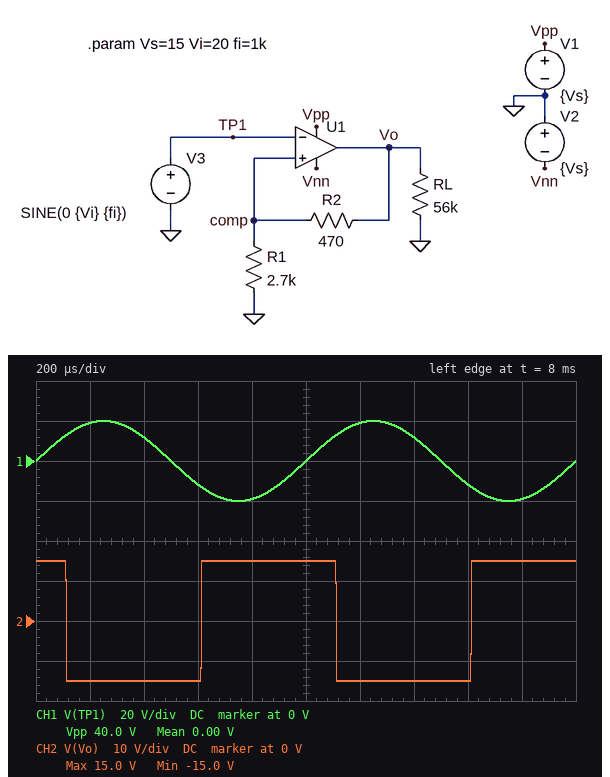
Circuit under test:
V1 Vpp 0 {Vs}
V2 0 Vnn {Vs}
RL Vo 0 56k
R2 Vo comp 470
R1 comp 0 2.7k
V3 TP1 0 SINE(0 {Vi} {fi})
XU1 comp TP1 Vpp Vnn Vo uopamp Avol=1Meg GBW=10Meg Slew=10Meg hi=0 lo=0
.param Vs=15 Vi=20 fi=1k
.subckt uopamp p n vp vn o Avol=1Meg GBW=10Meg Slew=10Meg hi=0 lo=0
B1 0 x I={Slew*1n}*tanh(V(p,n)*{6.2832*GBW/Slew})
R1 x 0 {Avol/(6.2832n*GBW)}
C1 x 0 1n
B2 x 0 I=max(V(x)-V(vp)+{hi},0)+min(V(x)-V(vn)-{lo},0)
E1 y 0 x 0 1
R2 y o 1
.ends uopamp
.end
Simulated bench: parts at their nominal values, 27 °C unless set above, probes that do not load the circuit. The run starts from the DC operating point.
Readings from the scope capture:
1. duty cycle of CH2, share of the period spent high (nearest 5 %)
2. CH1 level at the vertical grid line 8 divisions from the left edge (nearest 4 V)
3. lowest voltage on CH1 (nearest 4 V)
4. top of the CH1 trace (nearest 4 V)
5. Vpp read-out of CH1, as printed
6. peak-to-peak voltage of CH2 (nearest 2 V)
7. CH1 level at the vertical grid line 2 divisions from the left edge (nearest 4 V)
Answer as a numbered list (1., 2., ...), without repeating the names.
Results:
1. 50 %
2. -12 V
3. -20 V
4. 20 V
5. 40.0 V
6. 30 V
7. 12 V
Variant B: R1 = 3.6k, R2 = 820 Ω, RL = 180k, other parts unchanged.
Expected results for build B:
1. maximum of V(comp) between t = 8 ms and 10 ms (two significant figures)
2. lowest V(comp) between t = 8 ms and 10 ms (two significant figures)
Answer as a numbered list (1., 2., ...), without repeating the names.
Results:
1. 12 V
2. -12 V
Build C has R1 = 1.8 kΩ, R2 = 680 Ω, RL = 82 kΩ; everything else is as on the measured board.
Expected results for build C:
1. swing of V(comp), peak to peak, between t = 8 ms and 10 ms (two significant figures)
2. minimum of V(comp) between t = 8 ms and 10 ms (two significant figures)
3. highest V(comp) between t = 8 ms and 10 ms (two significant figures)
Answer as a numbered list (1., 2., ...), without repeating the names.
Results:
1. 22 V
2. -11 V
3. 11 V
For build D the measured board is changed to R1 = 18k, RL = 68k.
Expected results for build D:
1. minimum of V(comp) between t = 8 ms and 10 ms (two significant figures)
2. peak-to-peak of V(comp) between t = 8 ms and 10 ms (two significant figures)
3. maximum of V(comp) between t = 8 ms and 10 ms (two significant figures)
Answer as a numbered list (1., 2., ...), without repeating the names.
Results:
1. -15 V
2. 29 V
3. 15 V
